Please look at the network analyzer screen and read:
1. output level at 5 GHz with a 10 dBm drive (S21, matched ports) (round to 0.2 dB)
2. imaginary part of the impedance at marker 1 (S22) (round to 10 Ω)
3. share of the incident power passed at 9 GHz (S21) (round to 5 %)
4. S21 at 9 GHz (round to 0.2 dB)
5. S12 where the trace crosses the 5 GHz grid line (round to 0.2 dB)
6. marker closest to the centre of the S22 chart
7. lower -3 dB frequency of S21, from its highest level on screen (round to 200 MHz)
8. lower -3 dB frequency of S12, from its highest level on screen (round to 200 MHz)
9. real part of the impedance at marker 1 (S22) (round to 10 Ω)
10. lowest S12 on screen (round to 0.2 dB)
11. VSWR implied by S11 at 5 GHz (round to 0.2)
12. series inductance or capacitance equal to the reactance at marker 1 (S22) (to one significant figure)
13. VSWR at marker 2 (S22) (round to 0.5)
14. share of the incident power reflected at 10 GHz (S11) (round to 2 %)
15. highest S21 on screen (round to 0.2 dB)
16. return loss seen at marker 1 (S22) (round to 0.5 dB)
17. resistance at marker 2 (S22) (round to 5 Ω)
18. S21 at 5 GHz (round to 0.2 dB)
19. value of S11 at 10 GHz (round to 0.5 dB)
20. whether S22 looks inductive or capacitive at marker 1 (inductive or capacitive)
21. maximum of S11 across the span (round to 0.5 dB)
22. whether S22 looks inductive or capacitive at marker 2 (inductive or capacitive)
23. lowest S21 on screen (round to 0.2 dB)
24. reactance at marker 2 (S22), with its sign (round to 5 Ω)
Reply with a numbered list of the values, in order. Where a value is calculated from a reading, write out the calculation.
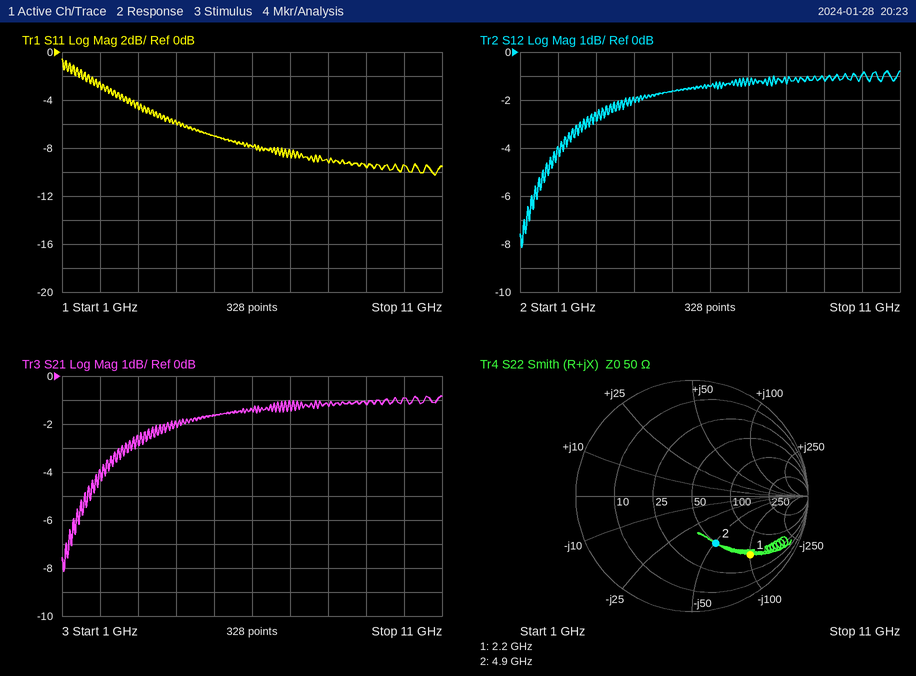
1. 10 dBm + (-1.6 dB) = 8.4 dBm
2. -100 Ω
3. 10^(-1.2/10) ≈ 75.9 %, so 75 % to the nearest 5 %
4. -1.2 dB
5. -1.6 dB
6. marker 2
7. 2.2 GHz
8. 2.2 GHz
9. 50 Ω
10. -8.2 dB
11. |Γ| = 10^(-7/20) = 0.4467; VSWR = (1 + 0.4467)/(1 − 0.4467) ≈ 2.6
12. C = 1/(2π × 2.2 GHz × 100 Ω) ≈ 723 fF, so 700 fF to one significant figure
13. 2.5
14. 10^(-9.5/10) ≈ 11.2 %, so 12 % to the nearest 2 %
15. -0.8 dB
16. 3.0 dB
17. 50 Ω
18. -1.6 dB
19. -9.5 dB
20. capacitive
21. -0.5 dB
22. capacitive
23. -8.2 dB
24. -50 Ω
